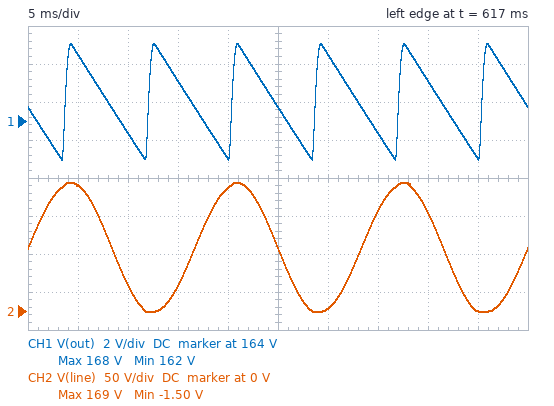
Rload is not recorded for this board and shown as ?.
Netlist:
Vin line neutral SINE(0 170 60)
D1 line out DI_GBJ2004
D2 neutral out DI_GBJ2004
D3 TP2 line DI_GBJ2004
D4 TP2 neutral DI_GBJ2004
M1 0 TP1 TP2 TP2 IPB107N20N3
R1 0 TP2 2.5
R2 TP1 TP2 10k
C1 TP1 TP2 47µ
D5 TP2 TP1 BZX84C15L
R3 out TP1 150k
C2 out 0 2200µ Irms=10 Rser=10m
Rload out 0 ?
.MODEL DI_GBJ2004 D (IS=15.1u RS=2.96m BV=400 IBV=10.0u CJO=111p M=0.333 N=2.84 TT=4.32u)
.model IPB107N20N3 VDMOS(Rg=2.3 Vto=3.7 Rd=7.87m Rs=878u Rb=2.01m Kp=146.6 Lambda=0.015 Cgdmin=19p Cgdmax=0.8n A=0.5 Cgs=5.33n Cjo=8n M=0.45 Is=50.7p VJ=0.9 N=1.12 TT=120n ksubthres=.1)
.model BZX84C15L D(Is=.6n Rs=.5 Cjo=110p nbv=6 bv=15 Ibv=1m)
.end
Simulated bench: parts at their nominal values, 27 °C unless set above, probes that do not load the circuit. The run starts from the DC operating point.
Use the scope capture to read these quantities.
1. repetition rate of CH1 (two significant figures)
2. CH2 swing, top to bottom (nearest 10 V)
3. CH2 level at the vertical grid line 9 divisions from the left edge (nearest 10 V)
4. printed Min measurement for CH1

120 Hz
170 V
0 V
162 V
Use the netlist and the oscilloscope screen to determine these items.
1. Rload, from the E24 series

91 Ω
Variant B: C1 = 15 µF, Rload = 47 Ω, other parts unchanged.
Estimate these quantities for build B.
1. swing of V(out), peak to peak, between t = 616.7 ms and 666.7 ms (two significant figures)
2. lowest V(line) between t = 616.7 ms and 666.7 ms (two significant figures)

11 V
-1.7 V
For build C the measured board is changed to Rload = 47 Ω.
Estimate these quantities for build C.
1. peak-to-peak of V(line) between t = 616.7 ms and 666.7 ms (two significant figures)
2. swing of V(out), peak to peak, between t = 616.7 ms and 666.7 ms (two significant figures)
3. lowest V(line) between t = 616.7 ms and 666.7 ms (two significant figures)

170 V
11 V
-1.7 V
